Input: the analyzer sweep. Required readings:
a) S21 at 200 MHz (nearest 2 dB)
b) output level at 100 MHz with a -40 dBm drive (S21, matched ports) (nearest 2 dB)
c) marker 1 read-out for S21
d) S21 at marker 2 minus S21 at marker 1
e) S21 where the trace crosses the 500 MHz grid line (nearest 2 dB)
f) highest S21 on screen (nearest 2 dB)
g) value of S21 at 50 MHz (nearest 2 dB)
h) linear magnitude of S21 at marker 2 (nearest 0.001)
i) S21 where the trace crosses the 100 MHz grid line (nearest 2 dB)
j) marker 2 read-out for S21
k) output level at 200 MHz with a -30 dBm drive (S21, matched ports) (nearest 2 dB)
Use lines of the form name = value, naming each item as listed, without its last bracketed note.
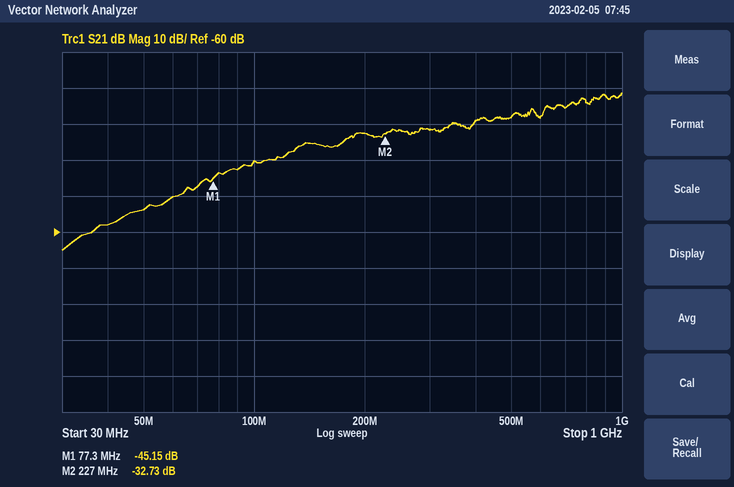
S21 at 200 MHz = -32 dB
output level at 100 MHz with a -40 dBm drive (S21, matched ports) = -80 dBm
marker 1 read-out for S21 = -45.15 dB
S21 at marker 2 minus S21 at marker 1 = 12.42 dB
S21 where the trace crosses the 500 MHz grid line = -28 dB
highest S21 on screen = -22 dB
value of S21 at 50 MHz = -54 dB
linear magnitude of S21 at marker 2 = 0.023
S21 where the trace crosses the 100 MHz grid line = -40 dB
marker 2 read-out for S21 = -32.73 dB
output level at 200 MHz with a -30 dBm drive (S21, matched ports) = -62 dBm
